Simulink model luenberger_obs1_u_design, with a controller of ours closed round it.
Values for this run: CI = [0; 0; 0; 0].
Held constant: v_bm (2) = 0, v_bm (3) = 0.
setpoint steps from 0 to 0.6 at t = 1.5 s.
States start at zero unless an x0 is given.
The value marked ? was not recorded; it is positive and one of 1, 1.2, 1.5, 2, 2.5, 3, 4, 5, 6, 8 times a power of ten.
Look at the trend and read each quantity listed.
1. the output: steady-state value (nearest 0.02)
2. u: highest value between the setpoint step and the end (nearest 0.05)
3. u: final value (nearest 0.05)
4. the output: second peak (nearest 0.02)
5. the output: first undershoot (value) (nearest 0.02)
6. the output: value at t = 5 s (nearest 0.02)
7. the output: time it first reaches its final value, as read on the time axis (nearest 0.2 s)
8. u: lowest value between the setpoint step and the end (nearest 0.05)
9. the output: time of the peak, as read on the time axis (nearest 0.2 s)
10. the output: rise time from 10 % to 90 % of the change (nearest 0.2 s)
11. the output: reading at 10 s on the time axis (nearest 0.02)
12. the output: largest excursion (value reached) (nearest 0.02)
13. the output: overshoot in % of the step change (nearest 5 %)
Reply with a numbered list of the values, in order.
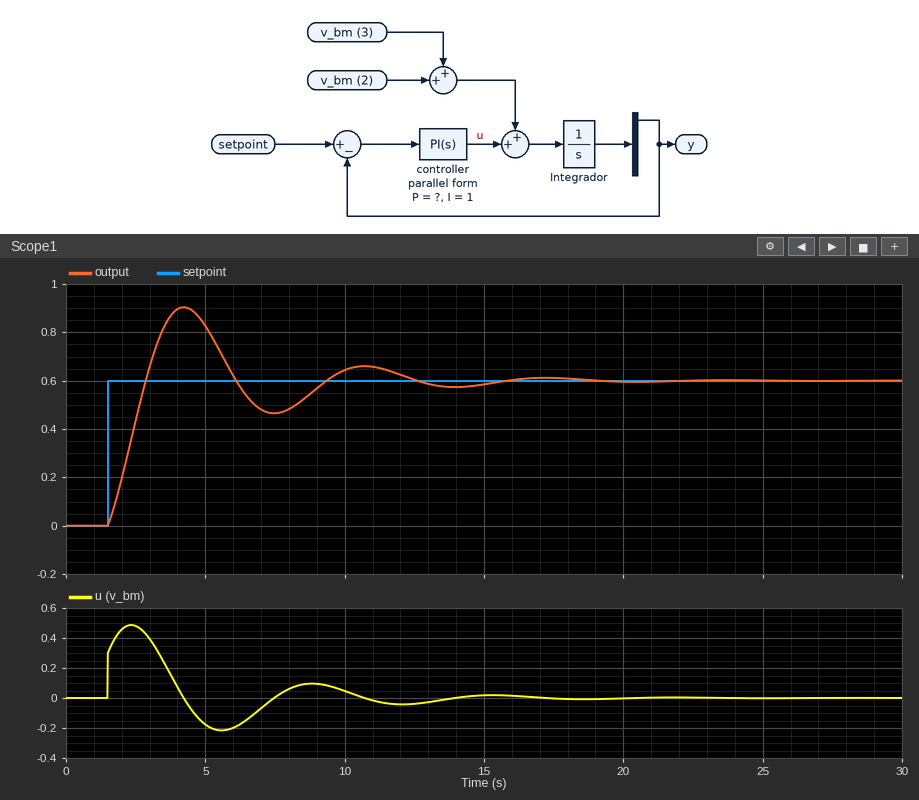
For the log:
1. 0.60
2. 0.50
3. 0.00
4. 0.66
5. 0.46
6. 0.82
7. 2.8 s
8. -0.20
9. 4.2 s
10. 1.0 s
11. 0.64
12. 0.90
13. 50 %
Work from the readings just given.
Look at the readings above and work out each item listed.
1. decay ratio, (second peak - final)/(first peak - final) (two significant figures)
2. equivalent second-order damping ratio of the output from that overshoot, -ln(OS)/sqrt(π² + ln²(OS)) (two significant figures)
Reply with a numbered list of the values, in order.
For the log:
1. 0.20
2. 0.22
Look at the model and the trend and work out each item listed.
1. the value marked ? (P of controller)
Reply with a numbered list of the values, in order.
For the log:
1. 0.5
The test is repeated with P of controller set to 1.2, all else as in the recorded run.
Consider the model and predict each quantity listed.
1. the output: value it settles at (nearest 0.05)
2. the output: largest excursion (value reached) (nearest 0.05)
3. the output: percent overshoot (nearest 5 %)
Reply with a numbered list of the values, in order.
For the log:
1. 0.60
2. 0.75
3. 25 %
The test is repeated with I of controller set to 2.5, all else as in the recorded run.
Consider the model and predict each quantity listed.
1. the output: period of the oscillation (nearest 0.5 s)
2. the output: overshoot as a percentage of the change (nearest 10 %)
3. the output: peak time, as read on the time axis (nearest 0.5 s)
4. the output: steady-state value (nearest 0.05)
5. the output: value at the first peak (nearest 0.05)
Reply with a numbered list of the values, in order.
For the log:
1. 4.0 s
2. 60 %
3. 3.5 s
4. 0.60
5. 1.00
